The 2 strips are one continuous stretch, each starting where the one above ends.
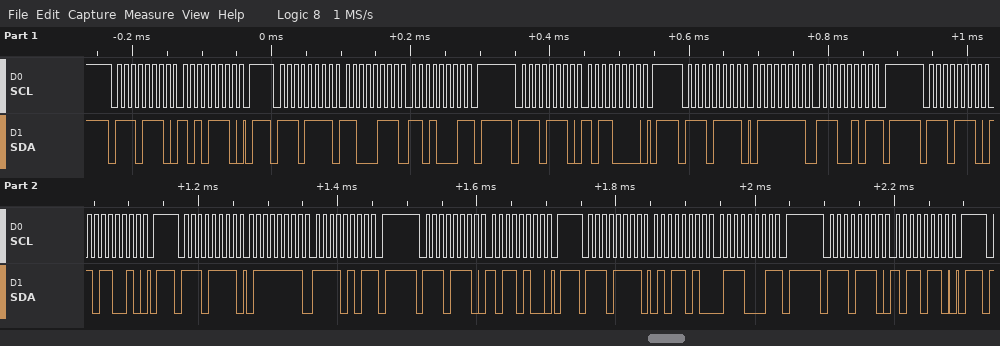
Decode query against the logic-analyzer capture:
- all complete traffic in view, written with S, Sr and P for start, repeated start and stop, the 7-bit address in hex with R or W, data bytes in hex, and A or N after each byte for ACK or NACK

S 77W A AE A P S 77R A C7 A D1 N P S 77W A B0 A P S 77R A 7F A E5 N P S 77W A B2 A P S 77R A 7F A F5 N P S 77W A B4 A P S 77R A 5A A 71 N P S 77W A B6 A P
